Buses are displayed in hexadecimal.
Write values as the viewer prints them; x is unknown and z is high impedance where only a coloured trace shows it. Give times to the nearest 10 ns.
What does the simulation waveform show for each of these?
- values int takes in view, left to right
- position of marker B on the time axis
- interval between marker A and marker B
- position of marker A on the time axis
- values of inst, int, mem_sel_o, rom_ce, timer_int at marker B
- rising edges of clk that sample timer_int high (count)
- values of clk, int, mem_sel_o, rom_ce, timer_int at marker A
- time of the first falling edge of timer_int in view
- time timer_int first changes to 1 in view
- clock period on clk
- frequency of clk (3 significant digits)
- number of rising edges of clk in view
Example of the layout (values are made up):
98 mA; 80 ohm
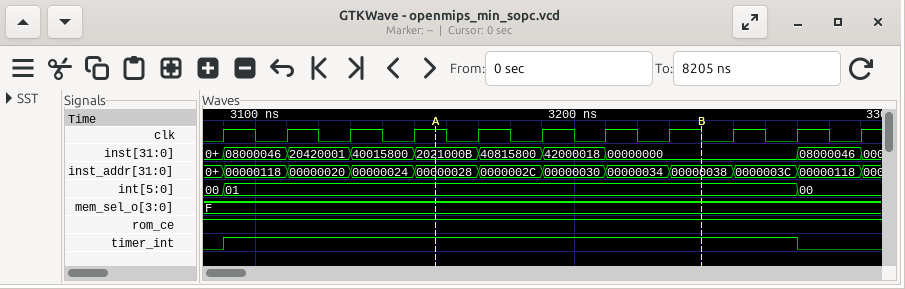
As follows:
00, 01, 00; 3240 ns; 80 ns; 3160 ns; inst=00000000, int=01, mem_sel_o=F, rom_ce=1, timer_int=1; 9; clk=1, int=01, mem_sel_o=F, rom_ce=1, timer_int=1; 3270 ns; 3090 ns; 20 ns; 50.0 MHz; 11
